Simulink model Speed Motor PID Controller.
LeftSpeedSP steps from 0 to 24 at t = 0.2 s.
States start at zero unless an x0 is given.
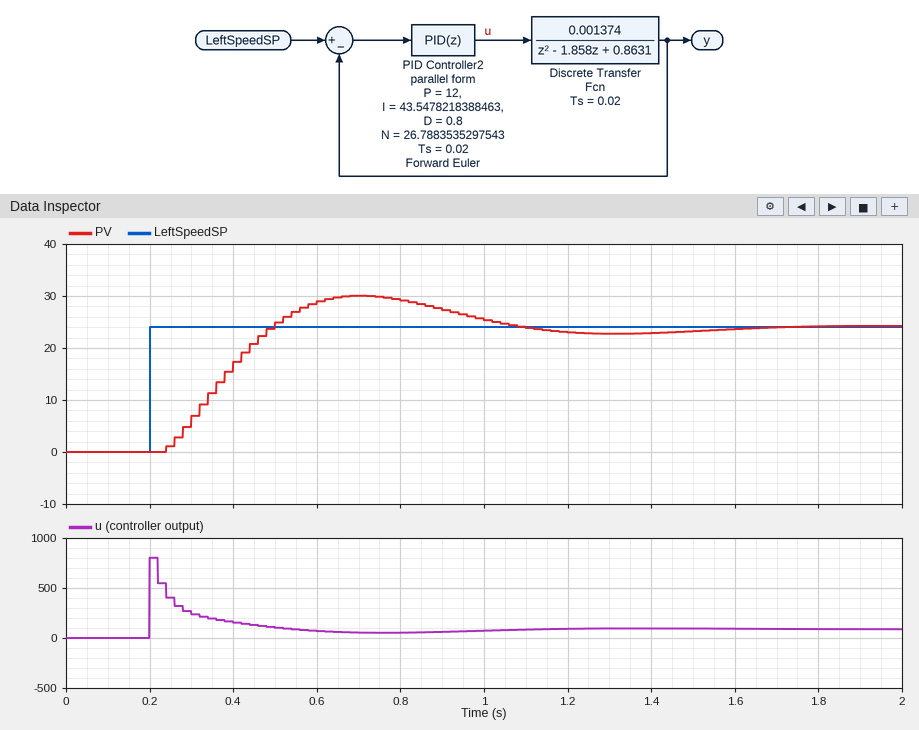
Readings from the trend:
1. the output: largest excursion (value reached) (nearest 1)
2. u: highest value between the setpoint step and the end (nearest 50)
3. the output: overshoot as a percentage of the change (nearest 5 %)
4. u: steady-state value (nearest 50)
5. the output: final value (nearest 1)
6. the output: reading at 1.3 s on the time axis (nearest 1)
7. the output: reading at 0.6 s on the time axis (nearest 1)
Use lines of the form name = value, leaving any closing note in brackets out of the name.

the output: largest excursion (value reached) = 30
u: highest value between the setpoint step and the end = 800
the output: overshoot as a percentage of the change = 25 %
u: steady-state value = 100
the output: final value = 24
the output: reading at 1.3 s on the time axis = 23
the output: reading at 0.6 s on the time axis = 29
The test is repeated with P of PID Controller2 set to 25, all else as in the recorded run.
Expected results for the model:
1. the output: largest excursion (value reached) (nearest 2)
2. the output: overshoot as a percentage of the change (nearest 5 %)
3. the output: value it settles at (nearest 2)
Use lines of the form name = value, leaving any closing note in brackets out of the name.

the output: largest excursion (value reached) = 32
the output: overshoot as a percentage of the change = 30 %
the output: value it settles at = 24
